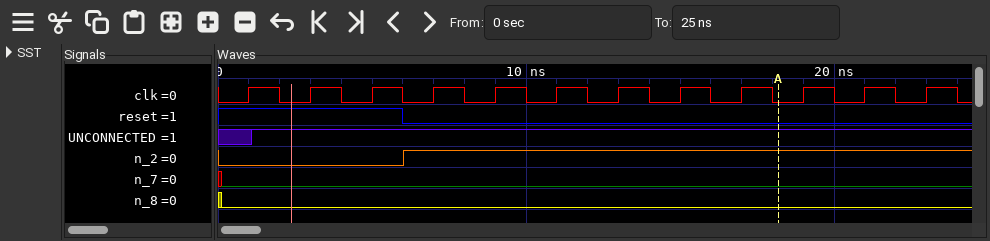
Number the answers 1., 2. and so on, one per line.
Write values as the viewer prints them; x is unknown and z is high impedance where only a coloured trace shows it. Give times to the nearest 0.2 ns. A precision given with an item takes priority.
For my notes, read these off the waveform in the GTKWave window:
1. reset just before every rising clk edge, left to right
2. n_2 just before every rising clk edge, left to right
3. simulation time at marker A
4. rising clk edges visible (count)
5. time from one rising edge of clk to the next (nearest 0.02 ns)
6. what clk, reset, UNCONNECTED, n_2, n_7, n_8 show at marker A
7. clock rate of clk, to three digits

1. 1 1 1 0 0 0 0 0 0 0 0 0
2. 0 0 0 1 1 1 1 1 1 1 1 1
3. 18.2 ns
4. 12
5. 2 ns
6. clk=0, reset=0, UNCONNECTED=1, n_2=1, n_7=0, n_8=0
7. 500 MHz
